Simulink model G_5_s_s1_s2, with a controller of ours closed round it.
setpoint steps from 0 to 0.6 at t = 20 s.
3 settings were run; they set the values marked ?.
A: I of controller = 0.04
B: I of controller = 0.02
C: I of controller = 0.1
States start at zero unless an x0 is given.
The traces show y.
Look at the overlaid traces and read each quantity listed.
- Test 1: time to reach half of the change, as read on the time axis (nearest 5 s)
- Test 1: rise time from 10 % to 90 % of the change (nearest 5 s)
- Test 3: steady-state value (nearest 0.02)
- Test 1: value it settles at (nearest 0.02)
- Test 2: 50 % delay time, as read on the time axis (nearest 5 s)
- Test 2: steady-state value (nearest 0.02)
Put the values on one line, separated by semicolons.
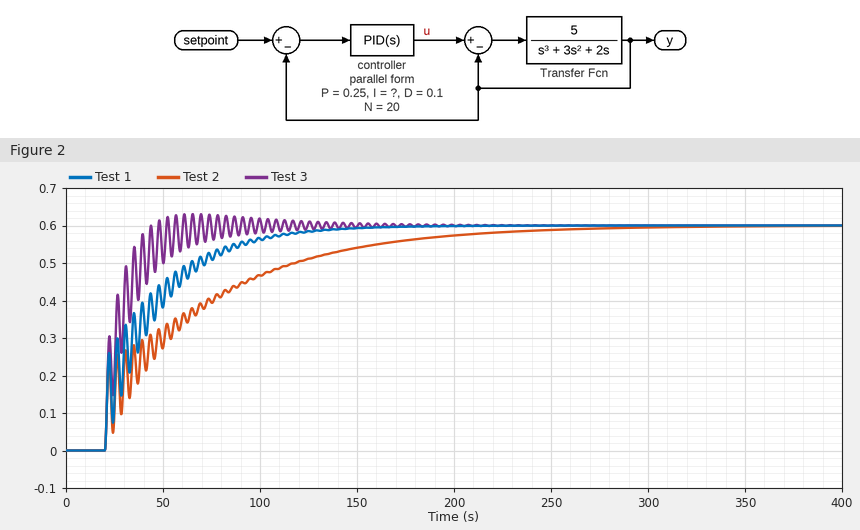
30 s; 60 s; 0.60; 0.60; 45 s; 0.60
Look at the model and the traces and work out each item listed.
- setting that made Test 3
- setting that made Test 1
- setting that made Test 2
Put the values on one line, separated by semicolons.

C; A; B
